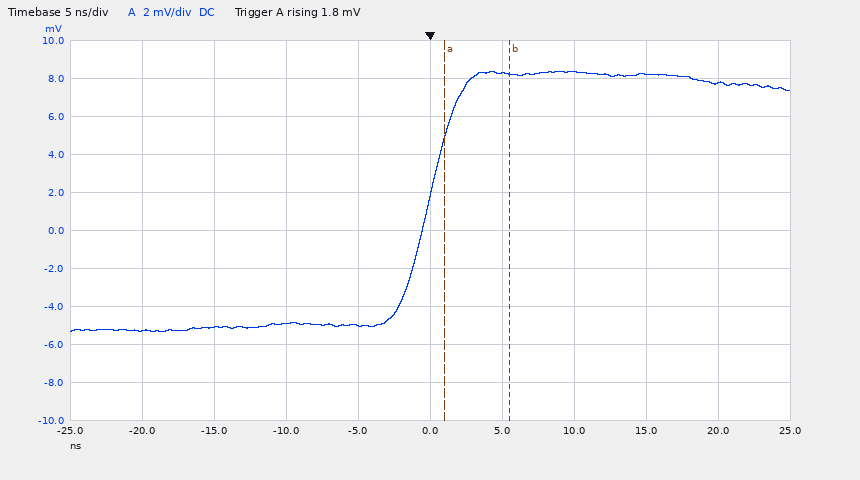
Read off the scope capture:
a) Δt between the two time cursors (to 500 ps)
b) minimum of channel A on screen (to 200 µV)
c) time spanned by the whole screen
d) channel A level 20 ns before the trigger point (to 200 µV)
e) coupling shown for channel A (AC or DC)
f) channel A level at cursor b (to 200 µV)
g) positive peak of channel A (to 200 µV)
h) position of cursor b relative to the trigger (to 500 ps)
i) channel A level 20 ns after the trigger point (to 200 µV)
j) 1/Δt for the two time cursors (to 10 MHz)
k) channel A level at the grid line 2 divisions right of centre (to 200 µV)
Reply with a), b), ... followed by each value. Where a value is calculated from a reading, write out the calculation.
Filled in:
a) 4.5 ns
b) -5.4 mV
c) 50 ns
d) -5.2 mV
e) DC
f) 8.2 mV
g) 8.4 mV
h) +5.5 ns
i) 7.8 mV
j) 1 / 4.5 ns ≈ 220 MHz
k) 8.4 mV
